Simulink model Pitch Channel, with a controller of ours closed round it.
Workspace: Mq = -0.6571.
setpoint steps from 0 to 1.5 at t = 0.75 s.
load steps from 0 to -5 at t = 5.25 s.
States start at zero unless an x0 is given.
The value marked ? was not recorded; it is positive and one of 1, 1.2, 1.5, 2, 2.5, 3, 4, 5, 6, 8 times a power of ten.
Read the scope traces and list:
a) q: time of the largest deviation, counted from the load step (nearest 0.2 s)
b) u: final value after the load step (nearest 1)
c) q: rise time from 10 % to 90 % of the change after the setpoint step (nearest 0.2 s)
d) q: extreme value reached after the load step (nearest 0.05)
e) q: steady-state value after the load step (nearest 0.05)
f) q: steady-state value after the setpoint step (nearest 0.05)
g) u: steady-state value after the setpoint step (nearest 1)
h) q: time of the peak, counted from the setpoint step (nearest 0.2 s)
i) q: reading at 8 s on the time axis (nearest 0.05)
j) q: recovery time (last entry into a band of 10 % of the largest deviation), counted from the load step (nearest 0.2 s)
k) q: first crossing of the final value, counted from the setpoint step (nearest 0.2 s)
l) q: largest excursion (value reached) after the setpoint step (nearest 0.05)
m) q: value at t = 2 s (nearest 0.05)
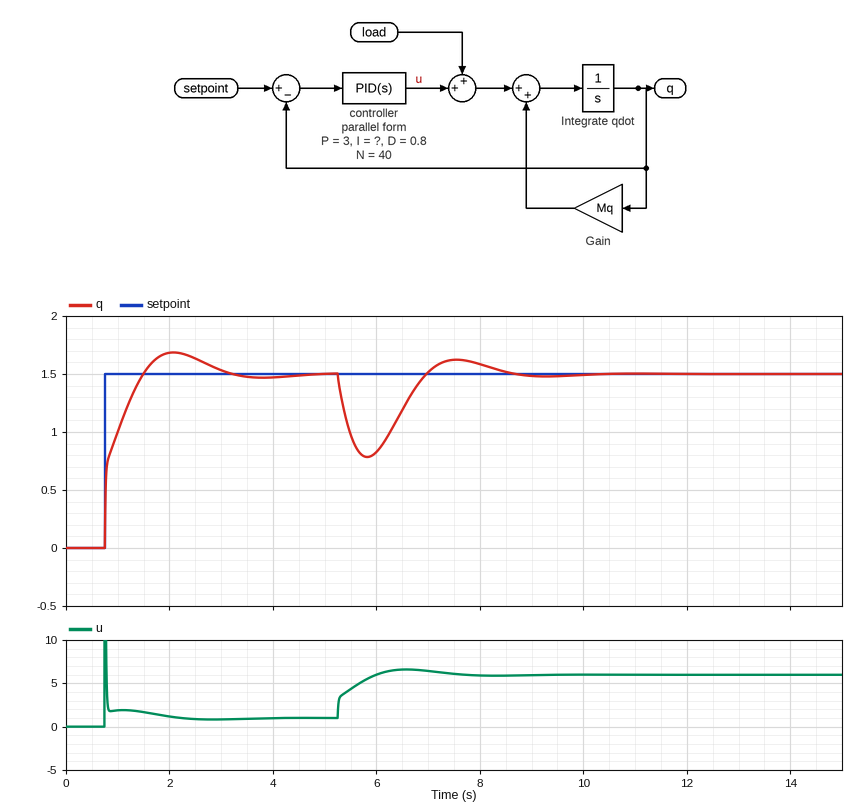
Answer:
0.6 s
6
0.6 s
0.80
1.50
1.50
1
1.4 s
1.60
2.8 s
0.8 s
1.70
1.70
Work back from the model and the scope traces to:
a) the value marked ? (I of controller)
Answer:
8
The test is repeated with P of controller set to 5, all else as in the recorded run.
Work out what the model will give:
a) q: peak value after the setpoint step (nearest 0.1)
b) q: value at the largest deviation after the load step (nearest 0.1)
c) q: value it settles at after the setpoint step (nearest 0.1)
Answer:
1.6
0.9
1.5
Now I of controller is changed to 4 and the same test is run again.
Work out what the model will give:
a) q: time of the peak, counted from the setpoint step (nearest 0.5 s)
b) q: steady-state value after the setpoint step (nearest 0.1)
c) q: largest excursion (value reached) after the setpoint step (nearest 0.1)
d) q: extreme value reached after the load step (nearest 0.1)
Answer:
2.0 s
1.5
1.6
0.6
